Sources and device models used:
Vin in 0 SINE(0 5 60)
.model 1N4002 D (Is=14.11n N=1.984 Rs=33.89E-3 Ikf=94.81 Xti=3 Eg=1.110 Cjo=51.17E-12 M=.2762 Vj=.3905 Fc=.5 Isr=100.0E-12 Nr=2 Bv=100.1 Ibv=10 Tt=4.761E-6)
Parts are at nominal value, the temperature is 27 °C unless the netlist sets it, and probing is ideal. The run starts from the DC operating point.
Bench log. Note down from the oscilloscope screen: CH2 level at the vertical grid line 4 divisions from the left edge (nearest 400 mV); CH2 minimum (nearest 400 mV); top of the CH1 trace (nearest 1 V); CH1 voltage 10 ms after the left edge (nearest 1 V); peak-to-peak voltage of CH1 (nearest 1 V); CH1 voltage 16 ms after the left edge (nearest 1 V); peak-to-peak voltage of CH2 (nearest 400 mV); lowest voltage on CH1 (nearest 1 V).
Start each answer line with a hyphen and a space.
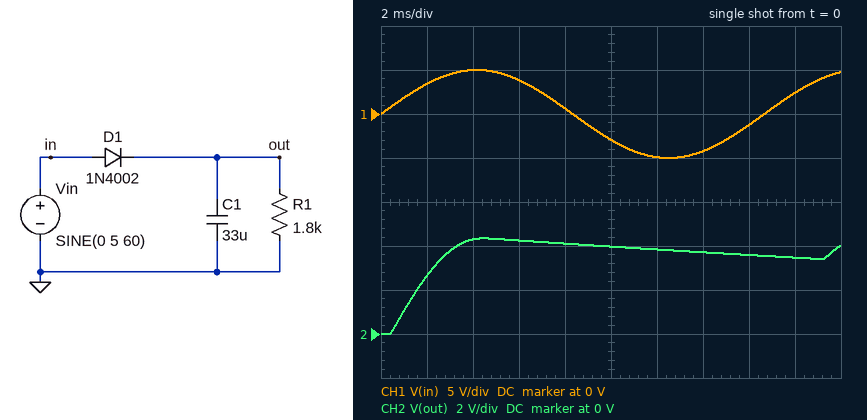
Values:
- 4.0 V
- 0 V
- 5 V
- -3 V
- 10 V
- -1 V
- 4.4 V
- -5 V
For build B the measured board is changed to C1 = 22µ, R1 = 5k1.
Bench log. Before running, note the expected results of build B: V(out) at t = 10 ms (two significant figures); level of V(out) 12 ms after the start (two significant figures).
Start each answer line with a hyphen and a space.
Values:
- 4.2 V
- 4.1 V
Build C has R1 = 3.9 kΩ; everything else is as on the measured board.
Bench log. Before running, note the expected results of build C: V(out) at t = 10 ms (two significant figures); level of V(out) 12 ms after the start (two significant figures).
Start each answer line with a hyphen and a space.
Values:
- 4.2 V
- 4.1 V
